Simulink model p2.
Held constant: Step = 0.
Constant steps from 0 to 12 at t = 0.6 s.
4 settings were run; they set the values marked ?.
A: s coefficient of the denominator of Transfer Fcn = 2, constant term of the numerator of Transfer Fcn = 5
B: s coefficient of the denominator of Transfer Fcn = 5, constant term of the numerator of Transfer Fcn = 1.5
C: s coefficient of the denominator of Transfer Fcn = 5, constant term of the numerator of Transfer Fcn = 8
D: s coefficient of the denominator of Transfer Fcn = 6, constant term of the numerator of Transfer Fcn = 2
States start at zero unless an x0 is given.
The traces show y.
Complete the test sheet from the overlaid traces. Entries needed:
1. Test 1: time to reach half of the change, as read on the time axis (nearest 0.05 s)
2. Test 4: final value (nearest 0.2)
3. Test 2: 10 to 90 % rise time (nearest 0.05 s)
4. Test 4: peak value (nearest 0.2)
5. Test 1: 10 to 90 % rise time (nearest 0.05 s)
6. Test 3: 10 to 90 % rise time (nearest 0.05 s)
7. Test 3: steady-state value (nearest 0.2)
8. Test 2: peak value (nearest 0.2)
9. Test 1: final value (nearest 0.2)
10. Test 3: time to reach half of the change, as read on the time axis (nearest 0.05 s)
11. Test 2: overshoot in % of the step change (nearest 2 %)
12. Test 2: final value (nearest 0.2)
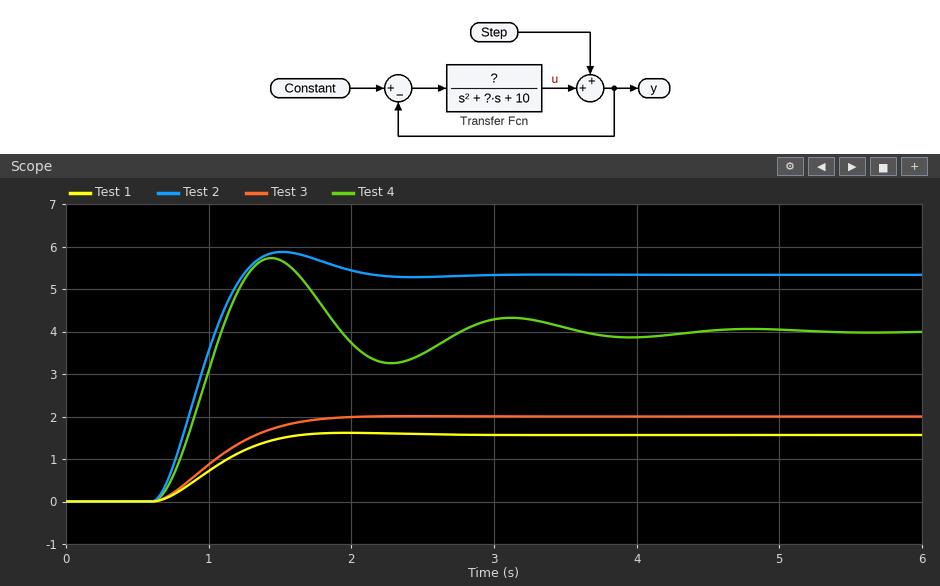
1.05 s
4.0
0.45 s
5.8
0.65 s
0.80 s
2.0
5.8
1.6
1.05 s
10 %
5.4
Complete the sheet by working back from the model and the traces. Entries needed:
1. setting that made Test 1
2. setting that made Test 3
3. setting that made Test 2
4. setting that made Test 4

B
D
C
A
